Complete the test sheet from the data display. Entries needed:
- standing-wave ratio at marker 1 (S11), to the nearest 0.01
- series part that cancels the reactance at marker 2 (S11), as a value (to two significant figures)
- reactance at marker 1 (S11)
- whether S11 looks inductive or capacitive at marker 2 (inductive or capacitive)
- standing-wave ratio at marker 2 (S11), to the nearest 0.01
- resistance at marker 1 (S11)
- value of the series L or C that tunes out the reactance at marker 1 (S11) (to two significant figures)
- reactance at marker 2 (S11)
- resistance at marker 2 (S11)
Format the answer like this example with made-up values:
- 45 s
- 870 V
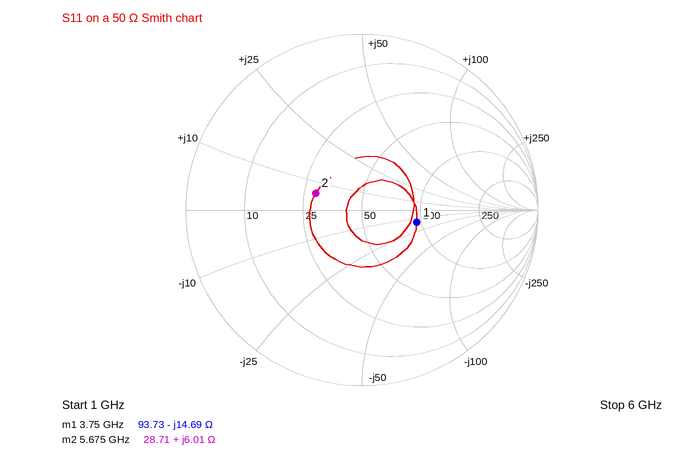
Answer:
- 1.94
- 4.7 pF
- -14.69 Ω
- inductive
- 1.78
- 93.73 Ω
- 620 pH
- +6.01 Ω
- 28.71 Ω
